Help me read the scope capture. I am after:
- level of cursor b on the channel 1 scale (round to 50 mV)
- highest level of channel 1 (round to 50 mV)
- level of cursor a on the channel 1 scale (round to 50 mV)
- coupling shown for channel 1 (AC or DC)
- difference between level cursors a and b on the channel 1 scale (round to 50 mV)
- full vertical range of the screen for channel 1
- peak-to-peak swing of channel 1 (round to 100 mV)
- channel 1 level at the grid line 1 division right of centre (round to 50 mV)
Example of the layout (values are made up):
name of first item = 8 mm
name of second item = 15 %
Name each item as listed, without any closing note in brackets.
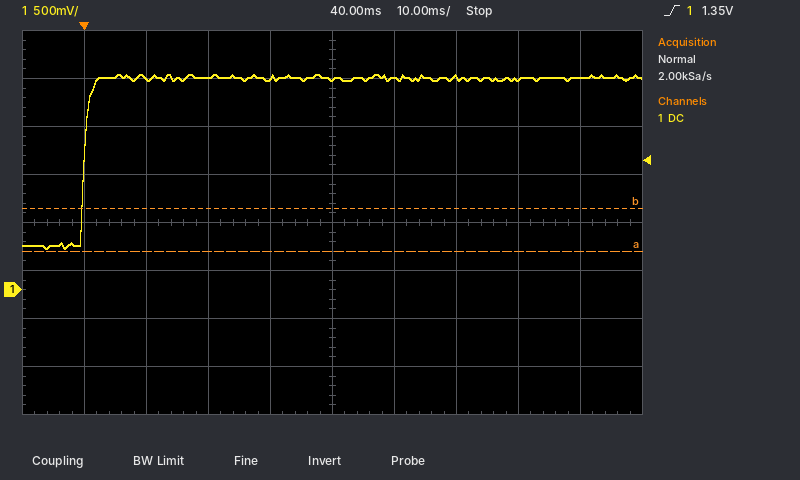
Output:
level of cursor b on the channel 1 scale = 850 mV
highest level of channel 1 = 2.25 V
level of cursor a on the channel 1 scale = 400 mV
coupling shown for channel 1 = DC
difference between level cursors a and b on the channel 1 scale = 450 mV
full vertical range of the screen for channel 1 = 4 V
peak-to-peak swing of channel 1 = 1.80 V
channel 1 level at the grid line 1 division right of centre = 2.20 V
